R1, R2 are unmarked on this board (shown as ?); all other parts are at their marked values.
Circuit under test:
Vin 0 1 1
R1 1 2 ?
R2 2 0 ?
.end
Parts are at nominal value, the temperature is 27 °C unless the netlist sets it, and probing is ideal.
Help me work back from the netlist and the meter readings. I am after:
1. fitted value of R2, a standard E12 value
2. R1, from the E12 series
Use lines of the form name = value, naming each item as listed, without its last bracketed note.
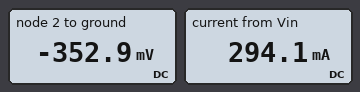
fitted value of R2, a standard E12 value = 1.2 Ω
R1, from the E12 series = 2.2 Ω
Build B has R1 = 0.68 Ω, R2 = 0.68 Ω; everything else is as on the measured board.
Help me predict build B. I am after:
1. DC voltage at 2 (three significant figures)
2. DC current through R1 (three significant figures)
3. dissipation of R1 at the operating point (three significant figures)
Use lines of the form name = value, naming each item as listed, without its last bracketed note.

DC voltage at 2 = -500 mV
DC current through R1 = 735 mA
dissipation of R1 at the operating point = 368 mW
